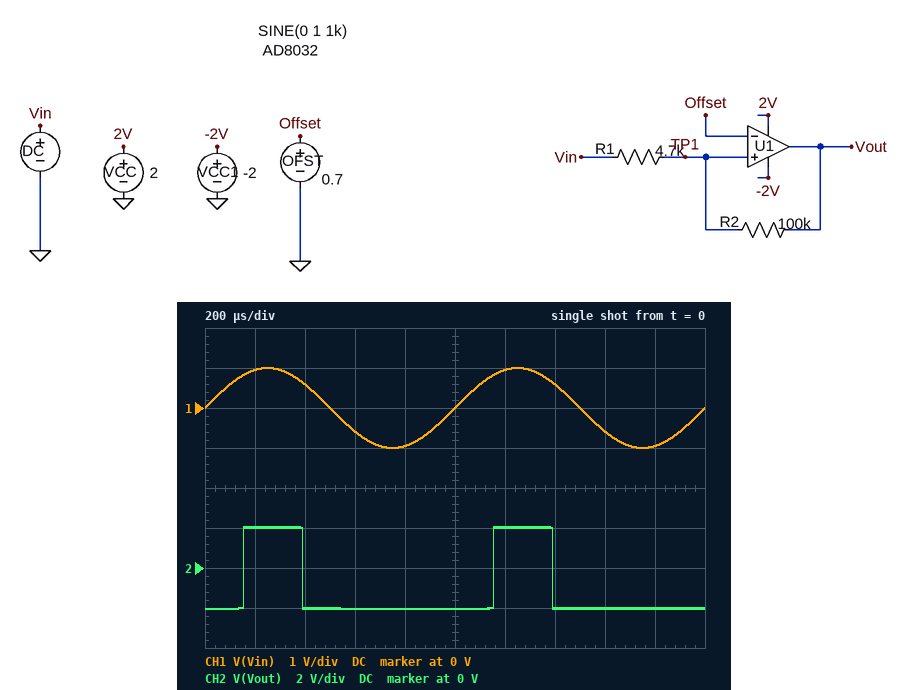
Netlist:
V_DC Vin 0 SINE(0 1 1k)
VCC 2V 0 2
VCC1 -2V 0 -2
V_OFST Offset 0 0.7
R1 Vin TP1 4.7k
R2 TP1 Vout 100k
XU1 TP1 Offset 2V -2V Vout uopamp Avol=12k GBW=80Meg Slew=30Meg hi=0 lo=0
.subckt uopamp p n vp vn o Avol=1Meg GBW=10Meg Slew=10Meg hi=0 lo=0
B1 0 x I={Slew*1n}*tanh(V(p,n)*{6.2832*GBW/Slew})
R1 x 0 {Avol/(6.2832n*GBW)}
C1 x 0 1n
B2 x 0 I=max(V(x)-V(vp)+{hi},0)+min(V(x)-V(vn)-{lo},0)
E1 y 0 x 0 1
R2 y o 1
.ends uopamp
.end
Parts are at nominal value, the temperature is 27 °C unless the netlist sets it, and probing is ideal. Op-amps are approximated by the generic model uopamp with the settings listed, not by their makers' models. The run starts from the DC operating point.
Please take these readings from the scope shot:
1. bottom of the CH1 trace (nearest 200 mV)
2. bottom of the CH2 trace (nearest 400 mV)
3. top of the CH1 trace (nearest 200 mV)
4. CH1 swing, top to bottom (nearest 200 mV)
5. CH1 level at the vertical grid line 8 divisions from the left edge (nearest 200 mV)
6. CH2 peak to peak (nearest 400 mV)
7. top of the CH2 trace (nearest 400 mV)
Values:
-1.0 V
-2.0 V
1.0 V
2.0 V
-600 mV
4.0 V
2.0 V
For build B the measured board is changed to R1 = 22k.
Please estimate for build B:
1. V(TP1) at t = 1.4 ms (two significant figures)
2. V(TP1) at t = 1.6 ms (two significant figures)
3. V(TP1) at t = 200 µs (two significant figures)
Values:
120 mV
-850 mV
410 mV
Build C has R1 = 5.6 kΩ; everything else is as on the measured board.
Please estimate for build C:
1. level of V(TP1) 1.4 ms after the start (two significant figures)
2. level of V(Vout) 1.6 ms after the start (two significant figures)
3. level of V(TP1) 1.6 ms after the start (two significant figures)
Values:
450 mV
-2.0 V
-660 mV
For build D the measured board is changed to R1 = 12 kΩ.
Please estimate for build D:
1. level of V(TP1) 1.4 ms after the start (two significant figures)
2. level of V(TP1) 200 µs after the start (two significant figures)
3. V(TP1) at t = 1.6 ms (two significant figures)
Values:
310 mV
630 mV
-740 mV
